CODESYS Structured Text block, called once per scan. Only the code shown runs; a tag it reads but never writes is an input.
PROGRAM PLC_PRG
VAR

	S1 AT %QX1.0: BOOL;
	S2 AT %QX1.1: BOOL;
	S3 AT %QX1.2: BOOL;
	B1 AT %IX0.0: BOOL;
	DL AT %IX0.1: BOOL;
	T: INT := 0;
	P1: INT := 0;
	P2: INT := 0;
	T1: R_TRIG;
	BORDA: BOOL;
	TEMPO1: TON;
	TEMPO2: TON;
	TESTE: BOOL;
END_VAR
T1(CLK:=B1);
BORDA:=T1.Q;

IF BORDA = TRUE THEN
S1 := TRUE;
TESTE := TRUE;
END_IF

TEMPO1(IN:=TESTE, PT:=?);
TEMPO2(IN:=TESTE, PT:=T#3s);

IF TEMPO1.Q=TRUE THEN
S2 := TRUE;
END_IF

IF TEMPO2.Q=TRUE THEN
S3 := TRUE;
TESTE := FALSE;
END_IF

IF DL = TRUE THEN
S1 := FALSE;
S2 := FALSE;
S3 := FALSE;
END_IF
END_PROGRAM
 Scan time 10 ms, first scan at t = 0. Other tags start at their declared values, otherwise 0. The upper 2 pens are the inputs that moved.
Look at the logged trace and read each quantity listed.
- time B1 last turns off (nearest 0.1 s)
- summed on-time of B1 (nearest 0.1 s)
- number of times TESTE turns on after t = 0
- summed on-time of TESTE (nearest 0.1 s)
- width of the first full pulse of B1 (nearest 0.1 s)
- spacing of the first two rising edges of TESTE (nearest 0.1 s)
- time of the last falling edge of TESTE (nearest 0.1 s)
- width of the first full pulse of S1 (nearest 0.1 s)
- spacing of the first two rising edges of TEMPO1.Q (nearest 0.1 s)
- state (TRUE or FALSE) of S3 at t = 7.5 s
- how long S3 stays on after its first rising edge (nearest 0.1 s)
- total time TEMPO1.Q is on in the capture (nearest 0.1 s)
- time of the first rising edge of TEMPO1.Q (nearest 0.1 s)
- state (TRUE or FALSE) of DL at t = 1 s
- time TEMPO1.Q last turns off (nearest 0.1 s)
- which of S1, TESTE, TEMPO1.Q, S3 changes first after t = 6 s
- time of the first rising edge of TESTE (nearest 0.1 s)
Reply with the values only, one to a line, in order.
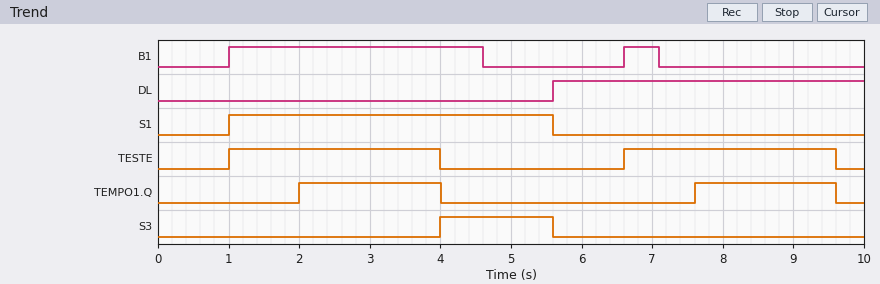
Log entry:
7.1 s
4.1 s
2
6.0 s
3.6 s
5.6 s
9.6 s
4.6 s
5.6 s
FALSE
1.6 s
4.0 s
2.0 s
FALSE
9.6 s
TESTE
1.0 s
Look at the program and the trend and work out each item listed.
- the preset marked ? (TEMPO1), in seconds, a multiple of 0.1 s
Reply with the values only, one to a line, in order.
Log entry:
1.0 s
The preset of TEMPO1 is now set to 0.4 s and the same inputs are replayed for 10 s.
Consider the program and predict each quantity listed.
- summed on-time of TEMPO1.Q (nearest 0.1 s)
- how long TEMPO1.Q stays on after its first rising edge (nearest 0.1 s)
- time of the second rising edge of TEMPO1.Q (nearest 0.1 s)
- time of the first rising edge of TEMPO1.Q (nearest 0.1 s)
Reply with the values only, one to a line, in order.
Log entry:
5.2 s
2.6 s
7.0 s
1.4 s
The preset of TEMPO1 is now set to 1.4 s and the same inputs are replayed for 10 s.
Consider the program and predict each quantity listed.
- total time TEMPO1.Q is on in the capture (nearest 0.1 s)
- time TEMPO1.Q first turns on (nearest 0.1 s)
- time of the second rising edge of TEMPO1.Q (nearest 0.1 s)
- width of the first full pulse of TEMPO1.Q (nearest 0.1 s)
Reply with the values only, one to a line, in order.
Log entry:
3.2 s
2.4 s
8.0 s
1.6 s
